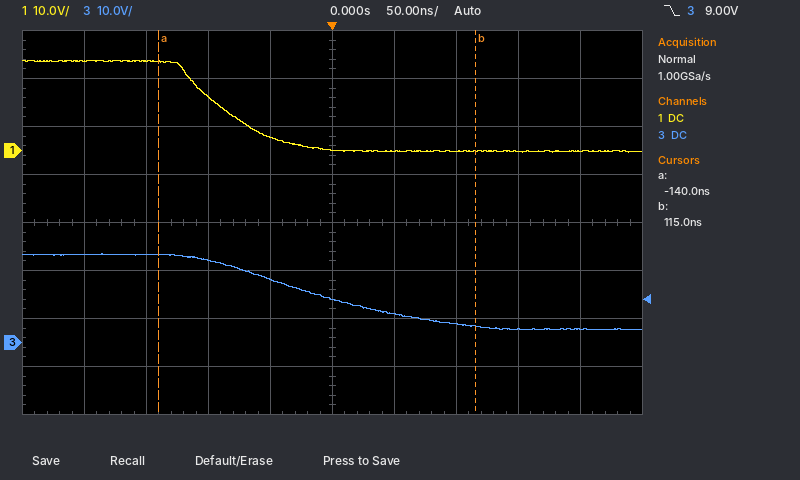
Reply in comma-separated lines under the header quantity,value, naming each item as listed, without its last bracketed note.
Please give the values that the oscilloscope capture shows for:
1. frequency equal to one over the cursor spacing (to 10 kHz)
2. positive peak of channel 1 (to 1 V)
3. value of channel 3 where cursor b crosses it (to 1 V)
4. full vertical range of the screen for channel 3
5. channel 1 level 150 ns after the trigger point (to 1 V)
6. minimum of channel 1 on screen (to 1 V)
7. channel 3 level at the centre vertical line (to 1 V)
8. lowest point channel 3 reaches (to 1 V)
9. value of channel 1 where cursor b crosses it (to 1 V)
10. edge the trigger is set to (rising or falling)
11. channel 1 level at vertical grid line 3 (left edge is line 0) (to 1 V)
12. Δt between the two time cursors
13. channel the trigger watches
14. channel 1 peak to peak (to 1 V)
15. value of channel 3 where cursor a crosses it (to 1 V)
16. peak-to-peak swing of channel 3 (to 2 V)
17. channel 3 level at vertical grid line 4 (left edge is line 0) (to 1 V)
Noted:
quantity,value
frequency equal to one over the cursor spacing,3.92 MHz
positive peak of channel 1,19 V
value of channel 3 where cursor b crosses it,3 V
full vertical range of the screen for channel 3,80 V
channel 1 level 150 ns after the trigger point,0 V
minimum of channel 1 on screen,0 V
channel 3 level at the centre vertical line,9 V
lowest point channel 3 reaches,3 V
value of channel 1 where cursor b crosses it,0 V
edge the trigger is set to,falling
channel 1 level at vertical grid line 3 (left edge is line 0),11 V
Δt between the two time cursors,255 ns
channel the trigger watches,channel 3
channel 1 peak to peak,19 V
value of channel 3 where cursor a crosses it,18 V
peak-to-peak swing of channel 3,16 V
channel 3 level at vertical grid line 4 (left edge is line 0),13 V
